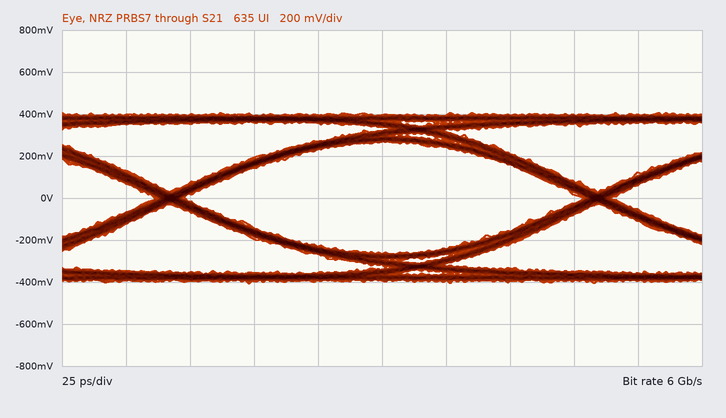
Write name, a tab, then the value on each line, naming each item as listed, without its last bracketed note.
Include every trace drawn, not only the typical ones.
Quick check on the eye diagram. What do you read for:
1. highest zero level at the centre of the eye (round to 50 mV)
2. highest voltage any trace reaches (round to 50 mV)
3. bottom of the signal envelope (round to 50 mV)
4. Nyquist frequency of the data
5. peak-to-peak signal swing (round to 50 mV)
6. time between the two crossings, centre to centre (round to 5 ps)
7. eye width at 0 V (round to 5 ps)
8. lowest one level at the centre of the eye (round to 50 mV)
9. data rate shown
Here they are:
highest zero level at the centre of the eye	-250 mV
highest voltage any trace reaches	400 mV
bottom of the signal envelope	-400 mV
Nyquist frequency of the data	3 GHz
peak-to-peak signal swing	800 mV
time between the two crossings, centre to centre	165 ps
eye width at 0 V	155 ps
lowest one level at the centre of the eye	250 mV
data rate shown	6 Gb/s
